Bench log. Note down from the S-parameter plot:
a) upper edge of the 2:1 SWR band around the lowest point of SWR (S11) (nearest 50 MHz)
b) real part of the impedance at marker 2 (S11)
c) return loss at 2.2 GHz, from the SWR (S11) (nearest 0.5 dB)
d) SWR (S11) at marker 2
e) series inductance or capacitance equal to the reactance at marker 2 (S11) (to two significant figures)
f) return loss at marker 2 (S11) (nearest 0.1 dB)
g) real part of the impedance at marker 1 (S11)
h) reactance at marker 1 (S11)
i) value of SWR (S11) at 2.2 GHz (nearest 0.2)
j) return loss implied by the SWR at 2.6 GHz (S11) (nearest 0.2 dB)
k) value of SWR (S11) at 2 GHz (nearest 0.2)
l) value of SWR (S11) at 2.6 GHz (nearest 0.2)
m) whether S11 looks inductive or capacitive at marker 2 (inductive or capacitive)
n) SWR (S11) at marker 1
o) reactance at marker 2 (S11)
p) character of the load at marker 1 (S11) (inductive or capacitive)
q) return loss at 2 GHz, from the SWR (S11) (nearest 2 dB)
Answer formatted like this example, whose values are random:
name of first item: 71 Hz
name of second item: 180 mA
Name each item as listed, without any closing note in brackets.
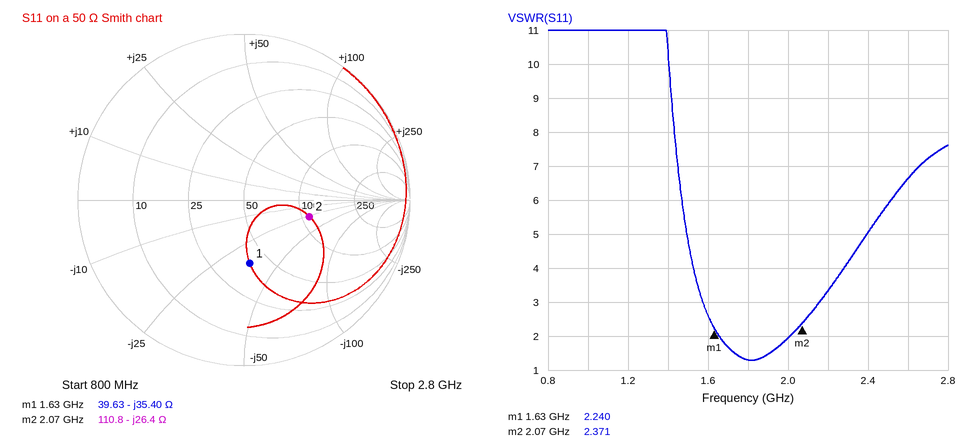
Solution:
upper edge of the 2:1 SWR band around the lowest point of SWR (S11): 2.00 GHz
real part of the impedance at marker 2: 110.8 Ω
return loss at 2.2 GHz, from the SWR (S11): 5.5 dB
SWR (S11) at marker 2: 2.371
series inductance or capacitance equal to the reactance at marker 2 (S11): 2.9 pF
return loss at marker 2 (S11): 7.8 dB
real part of the impedance at marker 1: 39.63 Ω
reactance at marker 1: -35.40 Ω
value of SWR (S11) at 2.2 GHz: 3.4
return loss implied by the SWR at 2.6 GHz (S11): 2.6 dB
value of SWR (S11) at 2 GHz: 2.0
value of SWR (S11) at 2.6 GHz: 6.6
whether S11 looks inductive or capacitive at marker 2: capacitive
SWR (S11) at marker 1: 2.240
reactance at marker 2: -26.4 Ω
character of the load at marker 1 (S11): capacitive
return loss at 2 GHz, from the SWR (S11): 10 dB
